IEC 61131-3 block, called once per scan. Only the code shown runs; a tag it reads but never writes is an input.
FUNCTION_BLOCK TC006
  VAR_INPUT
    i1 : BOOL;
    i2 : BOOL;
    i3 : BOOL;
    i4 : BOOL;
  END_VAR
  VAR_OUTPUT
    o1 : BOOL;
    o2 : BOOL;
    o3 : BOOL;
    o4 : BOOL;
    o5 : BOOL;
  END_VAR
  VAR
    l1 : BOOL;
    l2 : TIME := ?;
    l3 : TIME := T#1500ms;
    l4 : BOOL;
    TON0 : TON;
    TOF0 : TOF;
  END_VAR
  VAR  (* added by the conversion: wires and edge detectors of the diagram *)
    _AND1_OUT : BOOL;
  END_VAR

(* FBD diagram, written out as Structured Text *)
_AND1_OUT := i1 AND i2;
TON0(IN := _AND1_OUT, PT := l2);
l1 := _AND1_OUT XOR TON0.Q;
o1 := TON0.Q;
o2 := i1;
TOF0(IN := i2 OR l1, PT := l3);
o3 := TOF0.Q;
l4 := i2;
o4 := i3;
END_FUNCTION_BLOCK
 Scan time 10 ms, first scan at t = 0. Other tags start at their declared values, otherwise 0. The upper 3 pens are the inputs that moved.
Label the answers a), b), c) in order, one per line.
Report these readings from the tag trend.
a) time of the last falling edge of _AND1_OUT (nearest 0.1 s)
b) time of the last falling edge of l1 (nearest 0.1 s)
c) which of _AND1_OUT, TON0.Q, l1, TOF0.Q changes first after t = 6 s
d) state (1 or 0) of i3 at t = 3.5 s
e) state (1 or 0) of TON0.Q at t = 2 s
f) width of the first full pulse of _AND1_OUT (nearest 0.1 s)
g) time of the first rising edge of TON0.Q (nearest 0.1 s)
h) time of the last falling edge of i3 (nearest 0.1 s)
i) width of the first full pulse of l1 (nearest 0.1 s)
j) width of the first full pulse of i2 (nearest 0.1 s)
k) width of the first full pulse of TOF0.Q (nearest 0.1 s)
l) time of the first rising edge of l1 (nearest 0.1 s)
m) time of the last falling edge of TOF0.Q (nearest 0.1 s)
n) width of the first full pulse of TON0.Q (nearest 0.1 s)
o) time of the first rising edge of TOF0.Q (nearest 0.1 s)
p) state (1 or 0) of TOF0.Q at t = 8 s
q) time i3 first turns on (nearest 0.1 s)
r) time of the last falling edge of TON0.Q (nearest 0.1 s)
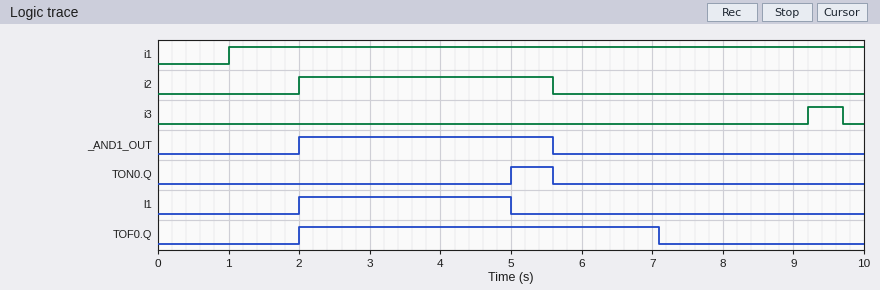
a) 5.6 s
b) 5.0 s
c) TOF0.Q
d) 0
e) 0
f) 3.6 s
g) 5.0 s
h) 9.7 s
i) 3.0 s
j) 3.6 s
k) 5.1 s
l) 2.0 s
m) 7.1 s
n) 0.6 s
o) 2.0 s
p) 0
q) 9.2 s
r) 5.6 s
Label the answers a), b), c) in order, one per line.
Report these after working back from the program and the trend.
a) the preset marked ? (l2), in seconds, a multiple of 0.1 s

a) 3.0 s
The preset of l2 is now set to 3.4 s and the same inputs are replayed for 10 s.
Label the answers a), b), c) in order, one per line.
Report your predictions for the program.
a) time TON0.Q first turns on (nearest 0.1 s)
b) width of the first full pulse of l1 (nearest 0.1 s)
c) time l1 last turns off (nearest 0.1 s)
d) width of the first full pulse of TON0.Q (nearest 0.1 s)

a) 5.4 s
b) 3.4 s
c) 5.4 s
d) 0.2 s
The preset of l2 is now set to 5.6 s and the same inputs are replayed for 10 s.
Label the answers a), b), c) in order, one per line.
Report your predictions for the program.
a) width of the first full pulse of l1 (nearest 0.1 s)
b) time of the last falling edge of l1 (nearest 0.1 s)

a) 3.6 s
b) 5.6 s
